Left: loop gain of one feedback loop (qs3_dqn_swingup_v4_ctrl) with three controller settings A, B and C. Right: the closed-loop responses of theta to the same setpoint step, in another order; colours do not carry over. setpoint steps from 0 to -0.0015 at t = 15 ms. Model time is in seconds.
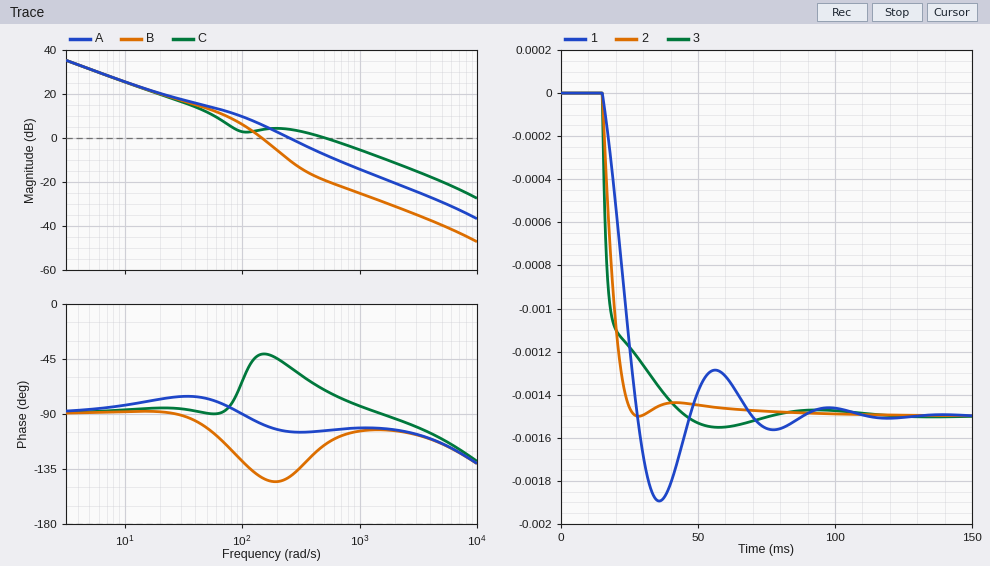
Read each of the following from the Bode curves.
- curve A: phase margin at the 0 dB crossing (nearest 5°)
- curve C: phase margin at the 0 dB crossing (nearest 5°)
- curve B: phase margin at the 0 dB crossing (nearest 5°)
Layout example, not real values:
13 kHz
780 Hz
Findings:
75°
110°
40°
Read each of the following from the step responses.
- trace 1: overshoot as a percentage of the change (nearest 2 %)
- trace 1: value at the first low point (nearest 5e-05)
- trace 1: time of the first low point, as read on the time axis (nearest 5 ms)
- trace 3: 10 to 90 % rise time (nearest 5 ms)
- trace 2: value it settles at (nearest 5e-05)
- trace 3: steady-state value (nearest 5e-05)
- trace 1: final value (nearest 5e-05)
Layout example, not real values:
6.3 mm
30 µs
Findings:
26 %
-0.00190
35 ms
20 ms
-0.00150
-0.00150
-0.00150
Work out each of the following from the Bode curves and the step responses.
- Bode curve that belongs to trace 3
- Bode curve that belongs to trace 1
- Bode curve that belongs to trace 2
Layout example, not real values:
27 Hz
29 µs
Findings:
C
B
A
